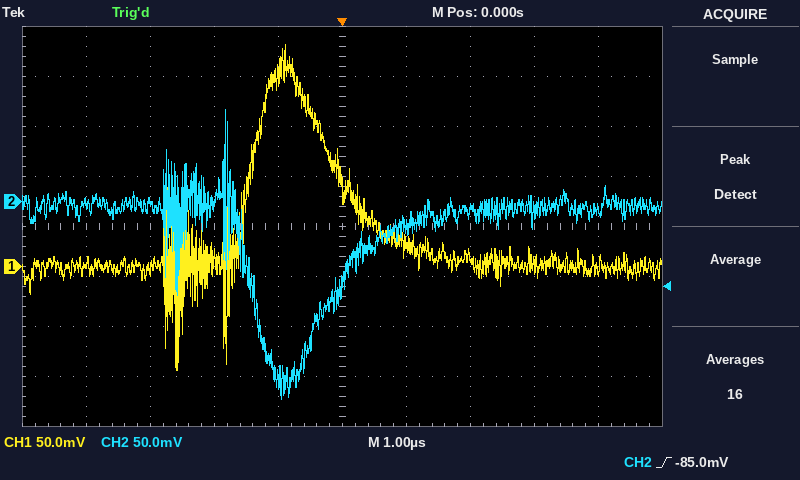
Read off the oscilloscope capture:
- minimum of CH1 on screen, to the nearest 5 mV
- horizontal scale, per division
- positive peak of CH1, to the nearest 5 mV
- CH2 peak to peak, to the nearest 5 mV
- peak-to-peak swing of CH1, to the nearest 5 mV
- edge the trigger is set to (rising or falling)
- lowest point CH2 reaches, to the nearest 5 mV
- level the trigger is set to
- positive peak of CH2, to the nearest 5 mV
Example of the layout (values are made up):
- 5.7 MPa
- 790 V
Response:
- -105 mV
- 1 µs
- 220 mV
- 290 mV
- 325 mV
- rising
- -200 mV
- -85.0 mV
- 90 mV
